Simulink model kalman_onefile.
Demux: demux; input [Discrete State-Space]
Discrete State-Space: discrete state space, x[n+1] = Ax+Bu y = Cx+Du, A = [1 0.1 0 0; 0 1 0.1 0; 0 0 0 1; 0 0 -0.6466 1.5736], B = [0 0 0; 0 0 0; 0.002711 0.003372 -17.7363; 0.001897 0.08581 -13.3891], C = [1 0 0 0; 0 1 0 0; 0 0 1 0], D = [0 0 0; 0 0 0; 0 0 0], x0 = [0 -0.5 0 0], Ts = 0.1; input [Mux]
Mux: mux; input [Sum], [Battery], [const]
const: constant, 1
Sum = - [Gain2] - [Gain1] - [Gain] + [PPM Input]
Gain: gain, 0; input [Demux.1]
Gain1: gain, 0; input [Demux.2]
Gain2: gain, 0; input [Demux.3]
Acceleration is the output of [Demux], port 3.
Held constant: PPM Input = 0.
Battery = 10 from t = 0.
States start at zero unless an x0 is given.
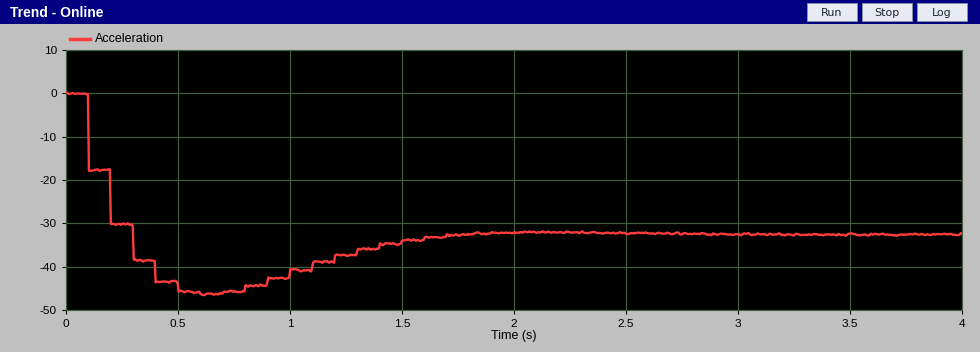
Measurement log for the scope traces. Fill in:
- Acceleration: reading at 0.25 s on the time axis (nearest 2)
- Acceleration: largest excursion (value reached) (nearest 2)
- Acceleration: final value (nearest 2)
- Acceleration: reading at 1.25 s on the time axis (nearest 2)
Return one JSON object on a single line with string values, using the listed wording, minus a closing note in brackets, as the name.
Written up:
{"Acceleration: reading at 0.25 s on the time axis": "-30", "Acceleration: largest excursion (value reached)": "-46", "Acceleration: final value": "-32", "Acceleration: reading at 1.25 s on the time axis": "-38"}
